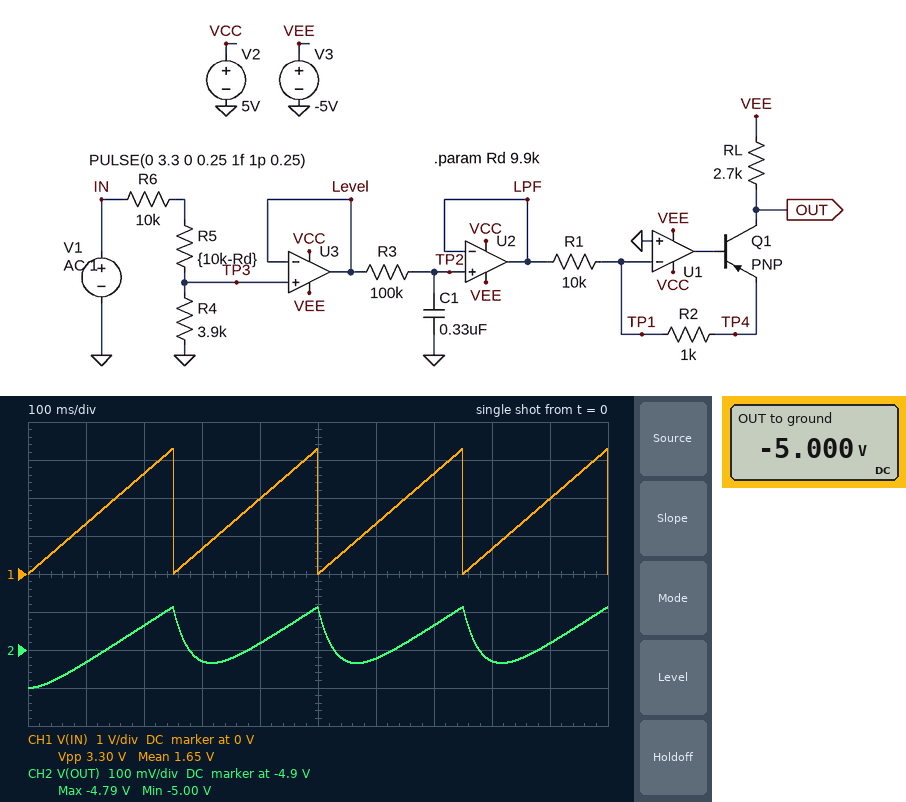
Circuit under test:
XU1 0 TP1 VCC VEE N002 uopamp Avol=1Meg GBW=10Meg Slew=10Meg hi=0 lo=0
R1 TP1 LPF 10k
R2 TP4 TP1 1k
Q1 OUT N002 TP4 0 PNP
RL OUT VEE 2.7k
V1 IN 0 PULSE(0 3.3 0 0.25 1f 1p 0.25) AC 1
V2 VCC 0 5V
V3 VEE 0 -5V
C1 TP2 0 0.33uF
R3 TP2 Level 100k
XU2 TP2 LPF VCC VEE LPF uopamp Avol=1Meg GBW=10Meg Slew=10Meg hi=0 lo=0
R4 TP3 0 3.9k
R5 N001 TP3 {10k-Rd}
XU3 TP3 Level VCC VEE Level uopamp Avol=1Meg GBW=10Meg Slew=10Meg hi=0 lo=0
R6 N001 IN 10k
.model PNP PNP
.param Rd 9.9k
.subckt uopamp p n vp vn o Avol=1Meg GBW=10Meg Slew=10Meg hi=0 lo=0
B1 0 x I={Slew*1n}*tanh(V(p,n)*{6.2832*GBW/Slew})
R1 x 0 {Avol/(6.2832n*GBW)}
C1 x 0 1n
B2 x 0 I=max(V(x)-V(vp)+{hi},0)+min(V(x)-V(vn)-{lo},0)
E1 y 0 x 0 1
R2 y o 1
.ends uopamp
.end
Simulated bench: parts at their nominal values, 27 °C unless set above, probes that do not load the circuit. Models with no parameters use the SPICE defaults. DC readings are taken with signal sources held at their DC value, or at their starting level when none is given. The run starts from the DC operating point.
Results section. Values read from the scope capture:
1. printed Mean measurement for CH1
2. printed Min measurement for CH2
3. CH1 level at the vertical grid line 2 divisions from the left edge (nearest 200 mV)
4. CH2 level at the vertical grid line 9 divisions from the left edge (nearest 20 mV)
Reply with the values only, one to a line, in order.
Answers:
1.65 V
-5.00 V
2.6 V
-4.88 V
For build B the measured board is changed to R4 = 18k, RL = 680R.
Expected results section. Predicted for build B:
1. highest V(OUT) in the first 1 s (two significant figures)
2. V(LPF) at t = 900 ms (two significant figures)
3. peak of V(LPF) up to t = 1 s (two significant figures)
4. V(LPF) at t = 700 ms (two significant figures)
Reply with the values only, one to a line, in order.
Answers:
-4.9 V
1.0 V
1.8 V
1.4 V
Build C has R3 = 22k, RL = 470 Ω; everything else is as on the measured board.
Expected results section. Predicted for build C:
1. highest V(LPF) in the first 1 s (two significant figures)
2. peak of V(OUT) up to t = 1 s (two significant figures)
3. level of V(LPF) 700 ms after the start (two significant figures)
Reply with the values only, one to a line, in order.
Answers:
890 mV
-5.0 V
710 mV
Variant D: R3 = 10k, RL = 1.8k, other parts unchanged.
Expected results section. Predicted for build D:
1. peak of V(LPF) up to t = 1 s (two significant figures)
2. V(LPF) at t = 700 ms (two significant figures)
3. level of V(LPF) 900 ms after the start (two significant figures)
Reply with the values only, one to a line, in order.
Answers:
910 mV
720 mV
540 mV
